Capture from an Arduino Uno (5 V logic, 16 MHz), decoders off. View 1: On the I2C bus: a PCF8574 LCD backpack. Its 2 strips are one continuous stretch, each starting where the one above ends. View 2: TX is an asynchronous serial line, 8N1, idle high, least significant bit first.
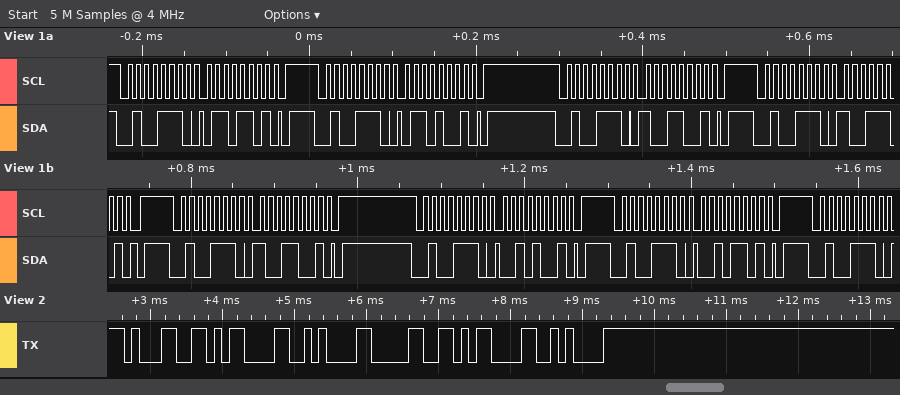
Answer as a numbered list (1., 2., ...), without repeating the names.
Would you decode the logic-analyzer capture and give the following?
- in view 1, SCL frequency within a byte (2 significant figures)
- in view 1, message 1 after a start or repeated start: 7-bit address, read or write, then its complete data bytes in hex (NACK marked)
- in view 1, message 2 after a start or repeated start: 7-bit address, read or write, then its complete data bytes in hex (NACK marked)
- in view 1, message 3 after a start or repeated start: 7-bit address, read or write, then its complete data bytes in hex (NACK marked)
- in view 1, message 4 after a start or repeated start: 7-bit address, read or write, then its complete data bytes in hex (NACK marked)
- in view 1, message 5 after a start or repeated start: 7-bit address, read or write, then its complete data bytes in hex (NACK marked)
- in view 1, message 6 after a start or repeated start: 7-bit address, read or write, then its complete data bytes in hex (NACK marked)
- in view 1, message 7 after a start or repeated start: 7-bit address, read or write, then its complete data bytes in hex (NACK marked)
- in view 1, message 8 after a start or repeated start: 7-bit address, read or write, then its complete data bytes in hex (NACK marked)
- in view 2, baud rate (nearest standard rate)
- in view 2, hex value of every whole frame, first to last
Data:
1. 100 kHz
2. 0x27 write: 6D
3. 0x27 write: 69
4. 0x27 write: 99
5. 0x27 write: 9D
6. 0x27 write: 99
7. 0x27 write: 29
8. 0x27 write: 2D
9. 0x27 write
10. 9600 baud
11. 31 0D 0A 30 0D 0A
